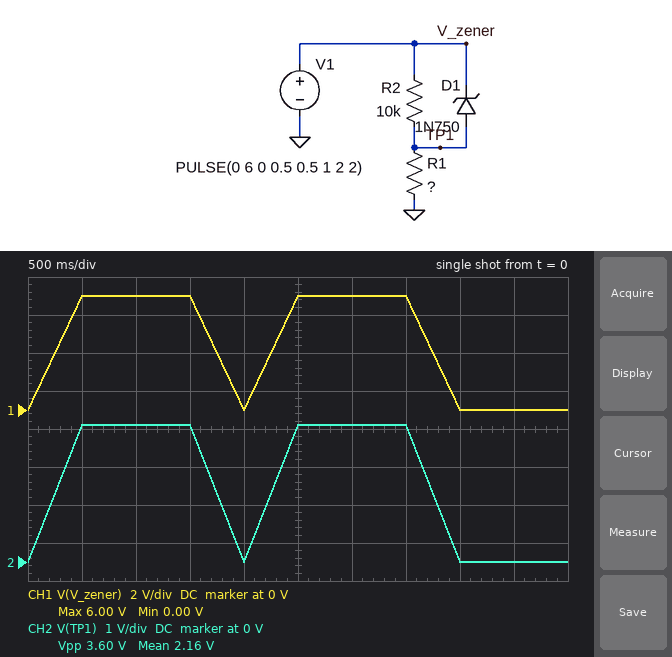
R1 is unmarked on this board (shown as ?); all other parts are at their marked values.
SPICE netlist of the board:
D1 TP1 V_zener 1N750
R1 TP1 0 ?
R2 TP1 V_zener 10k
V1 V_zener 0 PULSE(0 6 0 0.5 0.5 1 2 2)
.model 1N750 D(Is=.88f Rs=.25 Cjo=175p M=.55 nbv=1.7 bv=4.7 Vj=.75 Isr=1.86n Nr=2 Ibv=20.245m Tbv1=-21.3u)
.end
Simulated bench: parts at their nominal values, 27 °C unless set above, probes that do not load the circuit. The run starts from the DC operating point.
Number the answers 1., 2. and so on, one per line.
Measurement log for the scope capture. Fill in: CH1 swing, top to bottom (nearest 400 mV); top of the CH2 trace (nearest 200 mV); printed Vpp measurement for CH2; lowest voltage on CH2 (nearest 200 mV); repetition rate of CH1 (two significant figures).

1. 6.0 V
2. 3.6 V
3. 3.60 V
4. 0 V
5. 500 mHz
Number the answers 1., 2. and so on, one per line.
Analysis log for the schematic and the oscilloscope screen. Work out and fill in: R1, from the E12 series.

1. 15 kΩ
